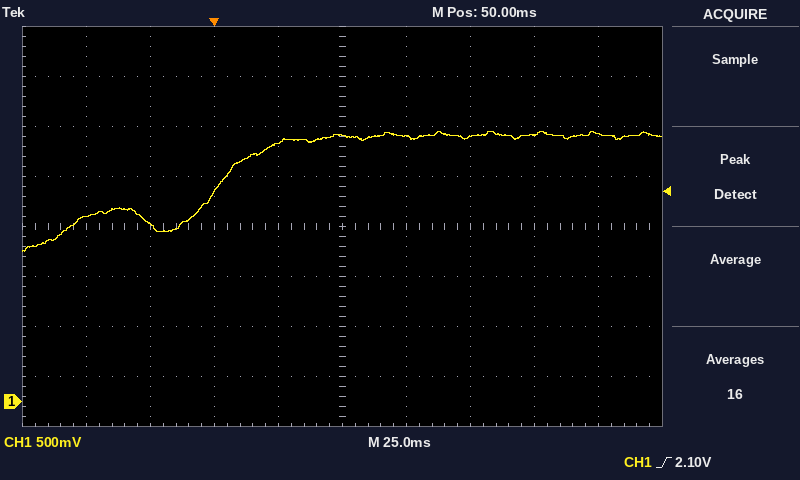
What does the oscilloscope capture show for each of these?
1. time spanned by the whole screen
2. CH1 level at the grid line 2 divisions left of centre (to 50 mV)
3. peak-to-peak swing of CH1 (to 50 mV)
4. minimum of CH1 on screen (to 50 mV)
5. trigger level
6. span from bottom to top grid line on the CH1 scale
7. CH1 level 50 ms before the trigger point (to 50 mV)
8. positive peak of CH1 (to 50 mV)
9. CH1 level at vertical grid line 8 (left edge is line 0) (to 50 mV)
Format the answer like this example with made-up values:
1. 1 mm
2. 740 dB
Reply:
1. 250 ms
2. 2.10 V
3. 1.20 V
4. 1.50 V
5. 2.10 V
6. 4 V
7. 1.85 V
8. 2.70 V
9. 2.65 V
